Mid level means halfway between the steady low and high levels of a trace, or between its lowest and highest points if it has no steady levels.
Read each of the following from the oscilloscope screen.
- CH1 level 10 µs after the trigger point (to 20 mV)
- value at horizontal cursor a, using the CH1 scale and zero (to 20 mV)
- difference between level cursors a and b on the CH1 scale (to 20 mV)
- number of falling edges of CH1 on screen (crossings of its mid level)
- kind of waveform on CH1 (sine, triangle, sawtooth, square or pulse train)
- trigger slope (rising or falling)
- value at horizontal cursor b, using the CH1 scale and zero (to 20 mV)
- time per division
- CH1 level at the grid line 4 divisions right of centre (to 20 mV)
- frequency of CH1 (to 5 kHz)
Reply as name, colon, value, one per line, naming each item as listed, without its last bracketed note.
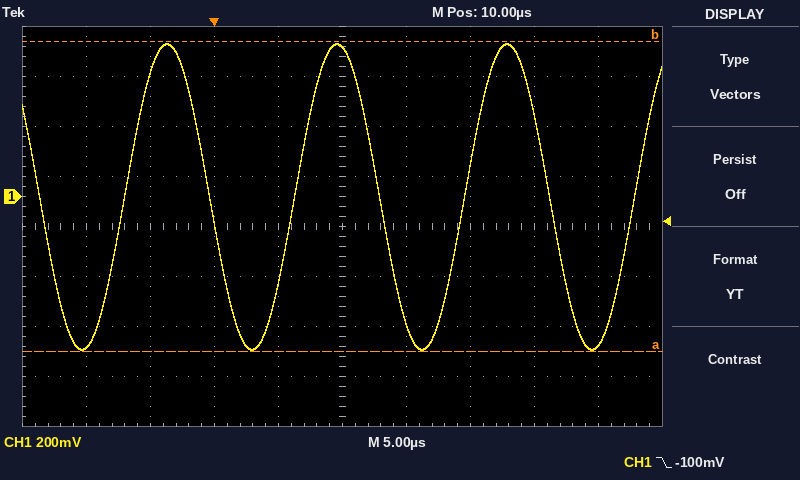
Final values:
CH1 level 10 µs after the trigger point: 600 mV
value at horizontal cursor a, using the CH1 scale and zero: -620 mV
difference between level cursors a and b on the CH1 scale: 1.24 V
number of falling edges of CH1 on screen: 4
kind of waveform on CH1: sine
trigger slope: falling
value at horizontal cursor b, using the CH1 scale and zero: 620 mV
time per division: 5 µs
CH1 level at the grid line 4 divisions right of centre: -600 mV
frequency of CH1: 75 kHz
